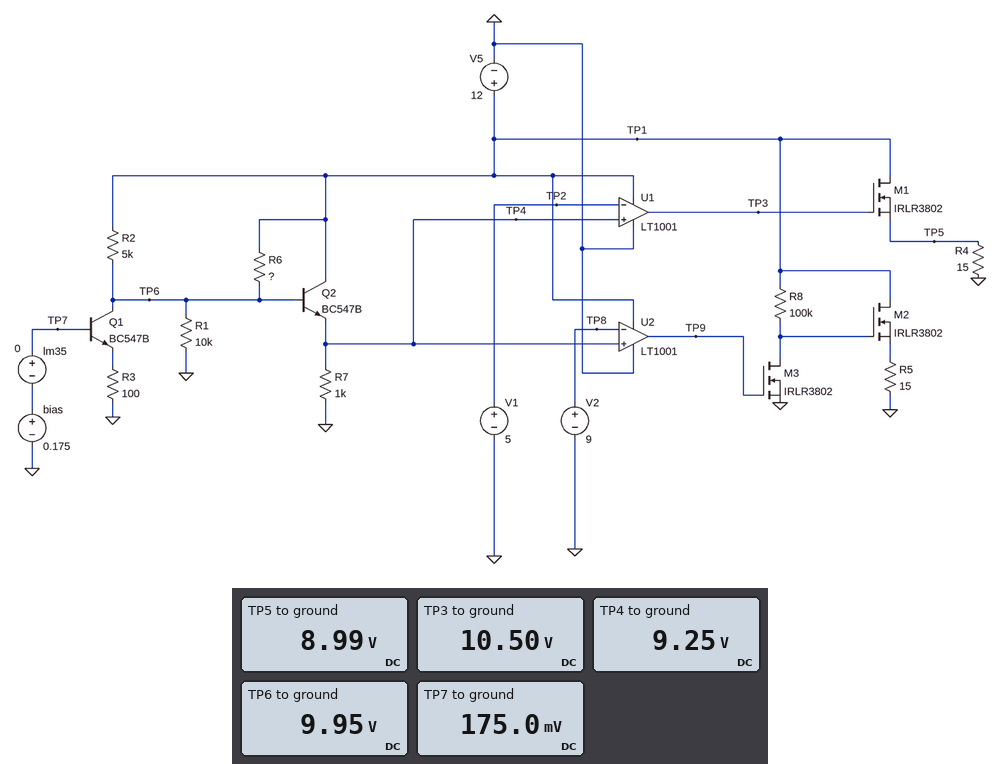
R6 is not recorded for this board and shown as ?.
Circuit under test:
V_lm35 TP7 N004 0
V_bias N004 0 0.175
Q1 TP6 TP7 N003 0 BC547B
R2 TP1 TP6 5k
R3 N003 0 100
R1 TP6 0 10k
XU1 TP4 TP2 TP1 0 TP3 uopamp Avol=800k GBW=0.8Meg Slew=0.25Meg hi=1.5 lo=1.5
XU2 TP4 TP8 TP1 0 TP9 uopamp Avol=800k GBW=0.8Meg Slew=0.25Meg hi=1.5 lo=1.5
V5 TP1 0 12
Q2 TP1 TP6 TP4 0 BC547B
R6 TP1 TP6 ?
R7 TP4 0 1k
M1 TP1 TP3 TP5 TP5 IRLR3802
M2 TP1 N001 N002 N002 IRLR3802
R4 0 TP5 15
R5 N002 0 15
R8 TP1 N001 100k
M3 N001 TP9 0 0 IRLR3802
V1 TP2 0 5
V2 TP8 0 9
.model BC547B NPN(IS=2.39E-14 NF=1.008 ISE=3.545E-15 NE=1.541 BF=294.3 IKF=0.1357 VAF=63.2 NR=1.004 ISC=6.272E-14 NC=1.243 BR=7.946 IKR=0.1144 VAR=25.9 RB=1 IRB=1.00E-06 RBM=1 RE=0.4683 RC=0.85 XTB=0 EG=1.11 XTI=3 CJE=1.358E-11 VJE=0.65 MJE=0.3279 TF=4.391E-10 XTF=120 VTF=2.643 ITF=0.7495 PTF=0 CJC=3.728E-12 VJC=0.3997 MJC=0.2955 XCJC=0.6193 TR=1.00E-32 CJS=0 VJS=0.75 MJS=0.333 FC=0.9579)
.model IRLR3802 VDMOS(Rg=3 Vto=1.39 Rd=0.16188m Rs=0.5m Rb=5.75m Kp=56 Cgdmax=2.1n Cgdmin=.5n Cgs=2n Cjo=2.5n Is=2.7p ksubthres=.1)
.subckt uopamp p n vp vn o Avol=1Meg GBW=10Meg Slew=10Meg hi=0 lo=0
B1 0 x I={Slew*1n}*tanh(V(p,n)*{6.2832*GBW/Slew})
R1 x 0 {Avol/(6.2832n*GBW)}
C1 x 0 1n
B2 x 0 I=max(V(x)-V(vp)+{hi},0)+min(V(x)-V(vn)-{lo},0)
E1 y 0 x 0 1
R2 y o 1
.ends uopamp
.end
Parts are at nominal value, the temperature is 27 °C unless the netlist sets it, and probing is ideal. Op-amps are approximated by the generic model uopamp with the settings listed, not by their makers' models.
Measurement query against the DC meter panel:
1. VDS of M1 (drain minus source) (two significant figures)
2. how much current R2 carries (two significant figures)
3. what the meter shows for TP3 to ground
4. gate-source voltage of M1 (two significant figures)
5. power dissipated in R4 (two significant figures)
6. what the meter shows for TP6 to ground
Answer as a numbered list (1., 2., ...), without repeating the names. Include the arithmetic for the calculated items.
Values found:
1. 12 V - 8.99 V = 3.0 V
2. (12 V - 9.95 V) / 5 kΩ = 410 µA
3. 10.50 V
4. 10.5 V - 8.99 V = 1.5 V
5. (8.99 V)^2 / 15 Ω = 5.4 W
6. 9.95 V
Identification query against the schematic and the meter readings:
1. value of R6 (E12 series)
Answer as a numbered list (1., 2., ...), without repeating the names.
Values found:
1. 3.3 kΩ
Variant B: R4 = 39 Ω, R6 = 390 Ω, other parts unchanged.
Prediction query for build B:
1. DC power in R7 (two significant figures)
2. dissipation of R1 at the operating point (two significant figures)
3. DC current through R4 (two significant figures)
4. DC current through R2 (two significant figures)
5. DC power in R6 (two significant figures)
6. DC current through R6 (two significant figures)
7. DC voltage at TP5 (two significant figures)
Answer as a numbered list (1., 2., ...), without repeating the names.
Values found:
1. 120 mW
2. 13 mW
3. 230 mA
4. 87 µA
5. 480 µW
6. 1.1 mA
7. 9.1 V
